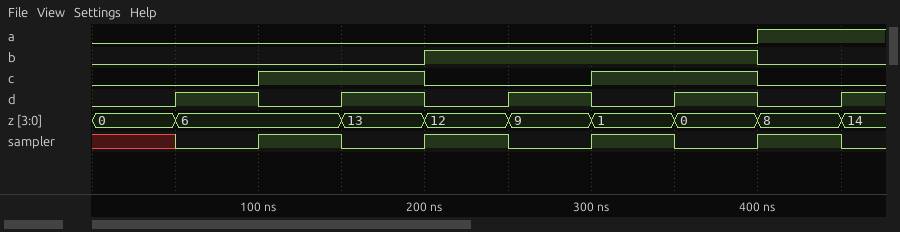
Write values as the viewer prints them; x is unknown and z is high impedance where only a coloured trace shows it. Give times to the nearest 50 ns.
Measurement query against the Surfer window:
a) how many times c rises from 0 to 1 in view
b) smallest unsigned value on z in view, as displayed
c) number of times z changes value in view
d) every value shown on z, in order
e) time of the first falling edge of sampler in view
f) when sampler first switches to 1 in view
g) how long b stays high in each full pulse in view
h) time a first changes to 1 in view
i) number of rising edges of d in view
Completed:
2
0
8
0, 6, 13, 12, 9, 1, 0, 8, 14
150 ns
100 ns
200 ns
400 ns
5
